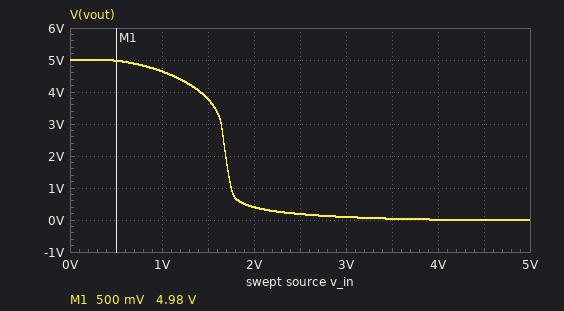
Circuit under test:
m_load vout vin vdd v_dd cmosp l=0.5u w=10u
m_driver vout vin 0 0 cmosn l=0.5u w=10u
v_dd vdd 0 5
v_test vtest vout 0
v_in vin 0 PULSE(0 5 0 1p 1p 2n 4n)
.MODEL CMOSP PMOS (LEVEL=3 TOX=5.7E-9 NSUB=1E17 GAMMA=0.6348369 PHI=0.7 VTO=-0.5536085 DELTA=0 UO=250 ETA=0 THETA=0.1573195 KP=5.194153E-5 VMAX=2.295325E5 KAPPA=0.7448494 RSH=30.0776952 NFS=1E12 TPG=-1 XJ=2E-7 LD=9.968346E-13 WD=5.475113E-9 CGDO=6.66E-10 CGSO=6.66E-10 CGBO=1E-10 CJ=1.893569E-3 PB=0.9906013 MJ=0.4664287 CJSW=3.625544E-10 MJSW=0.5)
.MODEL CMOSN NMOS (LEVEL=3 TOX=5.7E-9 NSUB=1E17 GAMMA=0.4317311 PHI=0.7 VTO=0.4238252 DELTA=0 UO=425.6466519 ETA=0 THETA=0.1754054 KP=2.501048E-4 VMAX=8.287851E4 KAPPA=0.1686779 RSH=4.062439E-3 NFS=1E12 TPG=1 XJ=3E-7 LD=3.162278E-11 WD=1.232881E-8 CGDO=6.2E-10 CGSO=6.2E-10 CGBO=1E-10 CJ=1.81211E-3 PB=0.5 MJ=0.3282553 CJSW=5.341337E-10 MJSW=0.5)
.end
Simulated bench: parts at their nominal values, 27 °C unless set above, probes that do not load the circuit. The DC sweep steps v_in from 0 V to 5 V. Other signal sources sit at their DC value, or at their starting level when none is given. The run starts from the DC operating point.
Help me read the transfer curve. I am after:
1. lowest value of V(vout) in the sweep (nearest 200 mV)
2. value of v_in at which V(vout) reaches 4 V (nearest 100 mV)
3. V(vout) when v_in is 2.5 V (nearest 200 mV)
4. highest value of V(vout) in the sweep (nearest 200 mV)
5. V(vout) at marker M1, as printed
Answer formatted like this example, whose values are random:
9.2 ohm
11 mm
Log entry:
0 V
1.4 V
200 mV
5.0 V
4.98 V
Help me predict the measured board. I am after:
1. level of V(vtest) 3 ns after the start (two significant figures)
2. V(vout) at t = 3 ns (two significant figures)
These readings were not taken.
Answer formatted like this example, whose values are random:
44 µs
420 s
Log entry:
5.0 V
5.0 V
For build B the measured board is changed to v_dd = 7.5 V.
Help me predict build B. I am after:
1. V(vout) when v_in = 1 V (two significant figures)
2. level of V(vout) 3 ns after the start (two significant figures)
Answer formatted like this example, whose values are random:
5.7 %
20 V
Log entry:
7.2 V
7.5 V
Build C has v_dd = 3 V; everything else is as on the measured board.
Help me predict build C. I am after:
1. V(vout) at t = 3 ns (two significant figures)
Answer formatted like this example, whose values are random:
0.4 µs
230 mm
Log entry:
3.0 V
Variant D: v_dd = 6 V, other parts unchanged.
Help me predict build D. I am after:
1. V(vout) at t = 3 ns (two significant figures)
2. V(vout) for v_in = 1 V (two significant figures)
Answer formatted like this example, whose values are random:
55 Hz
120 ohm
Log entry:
6.0 V
5.7 V
